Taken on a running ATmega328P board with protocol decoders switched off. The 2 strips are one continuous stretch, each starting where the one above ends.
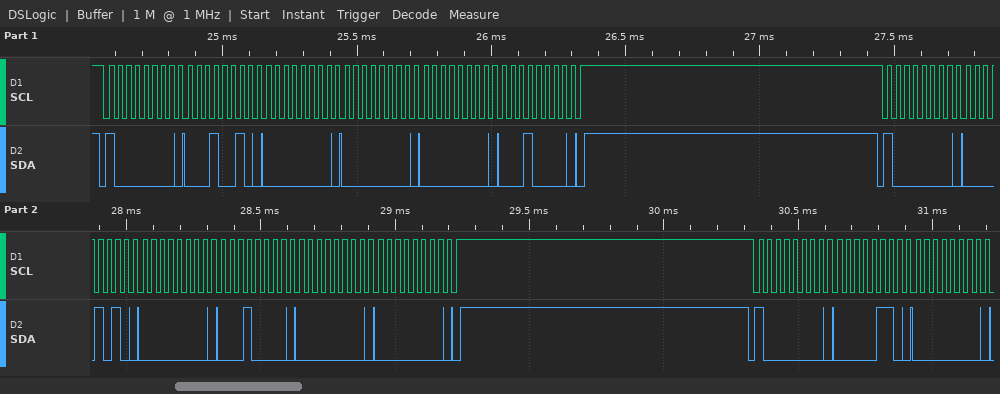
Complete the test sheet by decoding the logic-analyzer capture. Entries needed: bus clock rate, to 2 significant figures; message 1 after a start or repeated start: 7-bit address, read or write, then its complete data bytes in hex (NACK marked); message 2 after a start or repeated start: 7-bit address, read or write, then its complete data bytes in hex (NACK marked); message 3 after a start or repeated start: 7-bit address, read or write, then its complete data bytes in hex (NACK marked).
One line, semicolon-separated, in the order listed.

31 kHz; 0x40 write: 12 00 00 00 10; 0x40 write: 0A 00 10 00 00; 0x40 write: 06 00
